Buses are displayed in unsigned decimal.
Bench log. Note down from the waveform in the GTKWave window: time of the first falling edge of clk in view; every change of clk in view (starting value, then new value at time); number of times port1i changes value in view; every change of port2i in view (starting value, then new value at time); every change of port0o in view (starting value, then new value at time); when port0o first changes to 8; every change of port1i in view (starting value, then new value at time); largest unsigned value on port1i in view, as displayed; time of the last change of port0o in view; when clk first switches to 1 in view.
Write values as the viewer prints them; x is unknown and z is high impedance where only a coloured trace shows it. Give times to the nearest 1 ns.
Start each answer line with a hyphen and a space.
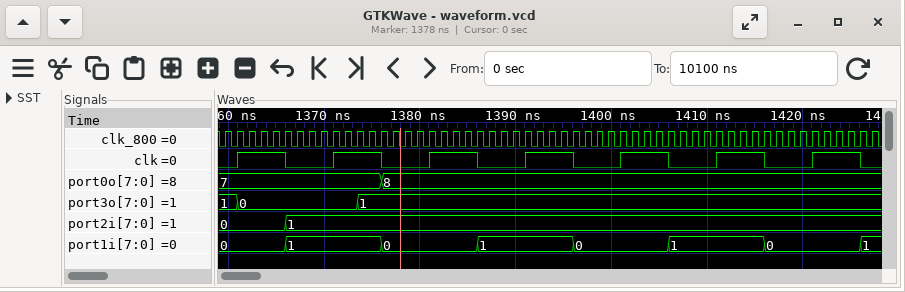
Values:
- 1366 ns
- 0, 1 at 1361 ns, 0 at 1366 ns, 1 at 1371 ns, 0 at 1376 ns, 1 at 1381 ns, 0 at 1386 ns, 1 at 1391 ns, 0 at 1396 ns, 1 at 1401 ns, 0 at 1406 ns, 1 at 1411 ns, 0 at 1416 ns, 1 at 1421 ns, 0 at 1426 ns
- 7
- 0, 1 at 1366 ns
- 7, 8 at 1376 ns
- 1376 ns
- 0, 1 at 1366 ns, 0 at 1376 ns, 1 at 1386 ns, 0 at 1396 ns, 1 at 1406 ns, 0 at 1416 ns, 1 at 1426 ns
- 1
- 1376 ns
- 1361 ns
